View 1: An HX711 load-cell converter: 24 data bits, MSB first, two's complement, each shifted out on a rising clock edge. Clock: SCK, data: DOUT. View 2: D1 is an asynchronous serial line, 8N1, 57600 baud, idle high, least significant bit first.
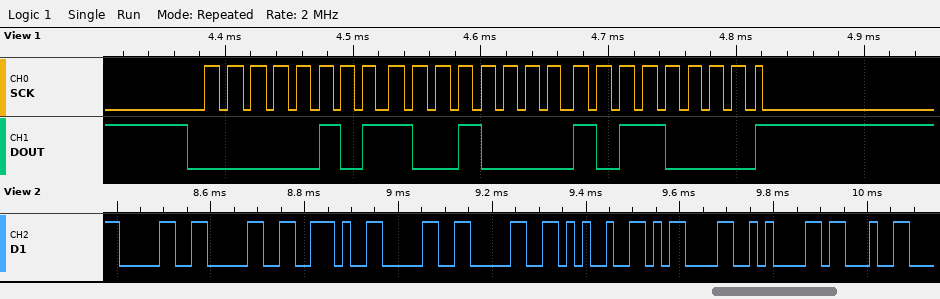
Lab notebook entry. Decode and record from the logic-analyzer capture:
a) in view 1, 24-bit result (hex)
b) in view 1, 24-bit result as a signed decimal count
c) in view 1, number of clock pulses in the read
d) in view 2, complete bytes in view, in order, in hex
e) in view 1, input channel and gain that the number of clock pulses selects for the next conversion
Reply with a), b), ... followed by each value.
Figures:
a) 0x0590B0
b) 364720
c) 25
d) 30 30 2E 30 30 25 0D 0A 23
e) channel A, gain 128
